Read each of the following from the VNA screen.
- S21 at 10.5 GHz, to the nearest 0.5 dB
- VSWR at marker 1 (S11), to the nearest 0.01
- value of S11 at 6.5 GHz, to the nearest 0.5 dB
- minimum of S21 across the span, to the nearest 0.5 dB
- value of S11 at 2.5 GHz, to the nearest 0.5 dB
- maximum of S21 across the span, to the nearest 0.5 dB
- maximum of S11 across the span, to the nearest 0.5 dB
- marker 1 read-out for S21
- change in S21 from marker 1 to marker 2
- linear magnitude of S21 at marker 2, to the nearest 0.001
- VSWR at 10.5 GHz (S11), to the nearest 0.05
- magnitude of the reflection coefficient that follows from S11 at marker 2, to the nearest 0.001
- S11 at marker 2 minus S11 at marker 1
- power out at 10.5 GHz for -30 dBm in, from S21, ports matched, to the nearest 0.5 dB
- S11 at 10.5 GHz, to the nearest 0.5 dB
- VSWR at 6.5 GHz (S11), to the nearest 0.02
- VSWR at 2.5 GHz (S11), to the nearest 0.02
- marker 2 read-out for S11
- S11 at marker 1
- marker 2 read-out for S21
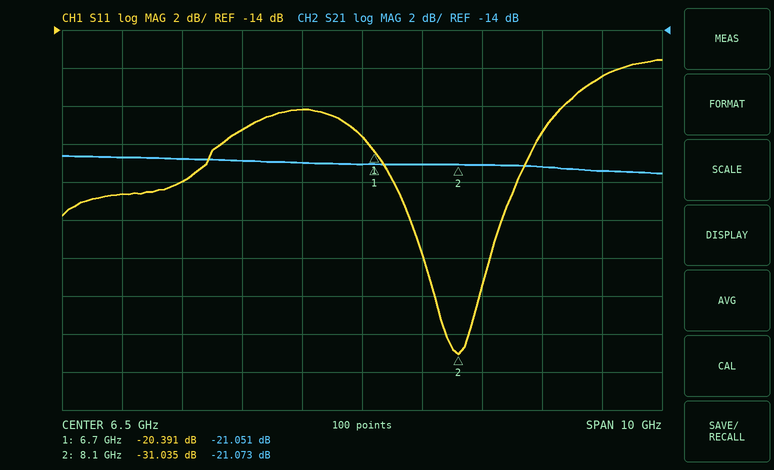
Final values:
-21.5 dB
1.21
-19.5 dB
-21.5 dB
-22.5 dB
-20.5 dB
-15.5 dB
-21.051 dB
-0.022 dB
0.088
1.35
0.028
-10.644 dB
-51.5 dBm
-16.5 dB
1.24
1.16
-31.035 dB
-20.391 dB
-21.073 dB
